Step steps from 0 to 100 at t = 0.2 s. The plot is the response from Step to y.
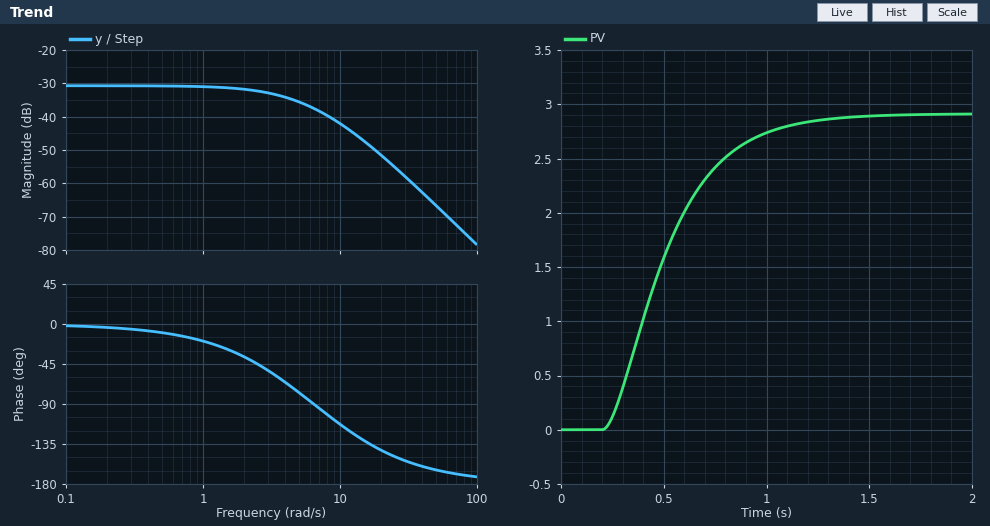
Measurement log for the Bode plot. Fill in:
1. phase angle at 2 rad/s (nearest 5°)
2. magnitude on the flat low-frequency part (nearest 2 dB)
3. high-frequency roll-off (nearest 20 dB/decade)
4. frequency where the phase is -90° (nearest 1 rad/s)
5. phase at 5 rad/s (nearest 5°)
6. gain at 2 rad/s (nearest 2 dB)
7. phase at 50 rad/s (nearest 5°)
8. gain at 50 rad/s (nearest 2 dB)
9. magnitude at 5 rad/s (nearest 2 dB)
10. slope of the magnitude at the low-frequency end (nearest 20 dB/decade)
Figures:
-35°
-30 dB
-40 dB/decade
6 rad/s
-75°
-32 dB
-165°
-66 dB
-36 dB
0 dB/decade
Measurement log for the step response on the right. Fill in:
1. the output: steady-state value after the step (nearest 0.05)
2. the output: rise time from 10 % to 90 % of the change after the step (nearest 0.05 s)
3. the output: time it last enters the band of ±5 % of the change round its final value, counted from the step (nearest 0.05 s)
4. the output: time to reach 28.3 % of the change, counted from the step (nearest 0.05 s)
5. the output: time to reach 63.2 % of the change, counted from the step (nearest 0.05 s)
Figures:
2.90
0.60 s
0.85 s
0.15 s
0.35 s
